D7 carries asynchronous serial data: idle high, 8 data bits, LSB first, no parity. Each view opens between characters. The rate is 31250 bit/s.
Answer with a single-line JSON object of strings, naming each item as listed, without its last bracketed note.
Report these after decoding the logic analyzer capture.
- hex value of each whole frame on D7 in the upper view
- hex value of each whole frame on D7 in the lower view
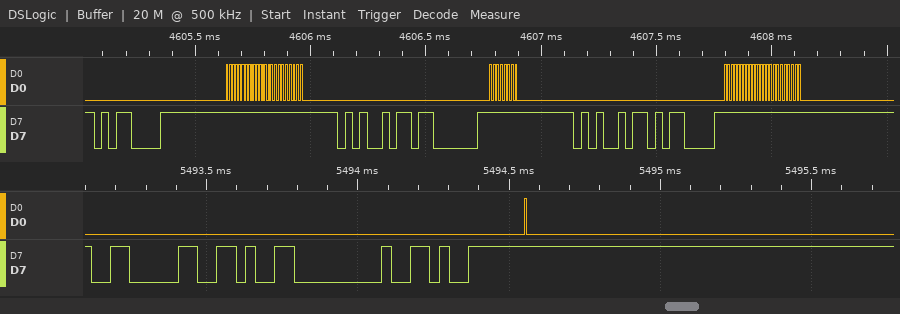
{"hex value of each whole frame on D7 in the upper view": "0D, A5, 03, A5, 0D", "hex value of each whole frame on D7 in the lower view": "06, 96, 00, 96"}
